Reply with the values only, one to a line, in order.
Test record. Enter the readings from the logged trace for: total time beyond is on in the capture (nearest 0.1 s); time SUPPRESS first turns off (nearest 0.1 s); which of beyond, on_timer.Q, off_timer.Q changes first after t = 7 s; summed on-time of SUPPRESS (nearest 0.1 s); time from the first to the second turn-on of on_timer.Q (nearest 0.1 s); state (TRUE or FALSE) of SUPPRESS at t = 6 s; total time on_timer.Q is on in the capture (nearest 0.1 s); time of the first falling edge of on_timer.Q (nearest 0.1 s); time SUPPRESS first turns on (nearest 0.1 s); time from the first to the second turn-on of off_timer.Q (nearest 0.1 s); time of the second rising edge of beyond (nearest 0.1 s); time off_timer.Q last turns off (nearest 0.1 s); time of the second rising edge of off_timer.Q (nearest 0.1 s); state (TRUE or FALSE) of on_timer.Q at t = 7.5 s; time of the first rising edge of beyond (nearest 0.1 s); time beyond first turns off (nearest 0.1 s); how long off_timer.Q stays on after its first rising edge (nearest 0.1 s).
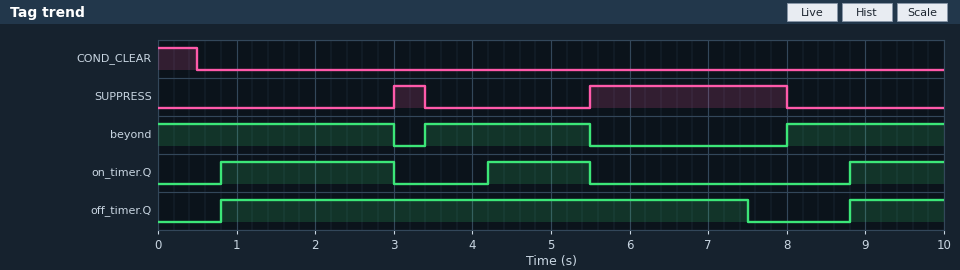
7.1 s
3.4 s
off_timer.Q
2.9 s
3.4 s
TRUE
4.7 s
3.0 s
3.0 s
8.0 s
8.0 s
7.5 s
8.8 s
FALSE
3.4 s
3.0 s
6.7 s
